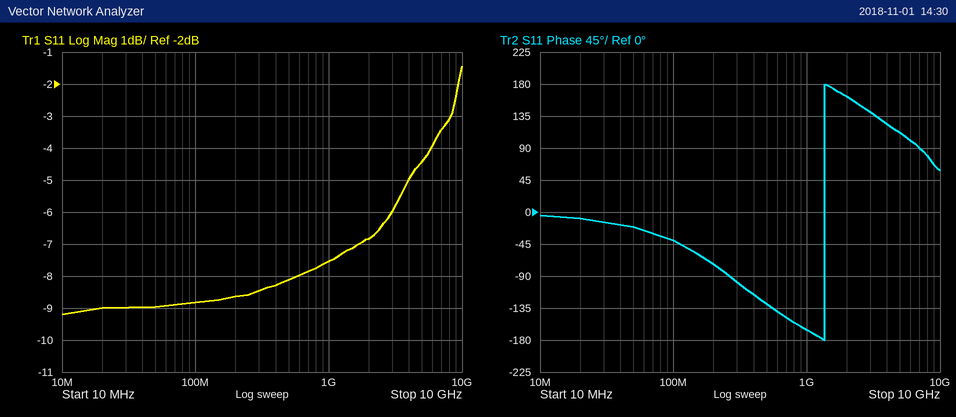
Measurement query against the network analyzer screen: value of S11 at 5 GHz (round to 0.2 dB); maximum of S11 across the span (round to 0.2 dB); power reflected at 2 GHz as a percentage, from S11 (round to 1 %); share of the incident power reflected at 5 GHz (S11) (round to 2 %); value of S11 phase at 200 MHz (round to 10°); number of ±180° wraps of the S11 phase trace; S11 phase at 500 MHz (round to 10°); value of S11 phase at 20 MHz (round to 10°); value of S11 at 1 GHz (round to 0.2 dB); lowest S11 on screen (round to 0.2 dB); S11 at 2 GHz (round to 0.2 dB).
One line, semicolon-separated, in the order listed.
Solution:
-4.4 dB; -1.4 dB; 21 %; 36 %; -70°; 1; -130°; -10°; -7.6 dB; -9.2 dB; -6.8 dB
